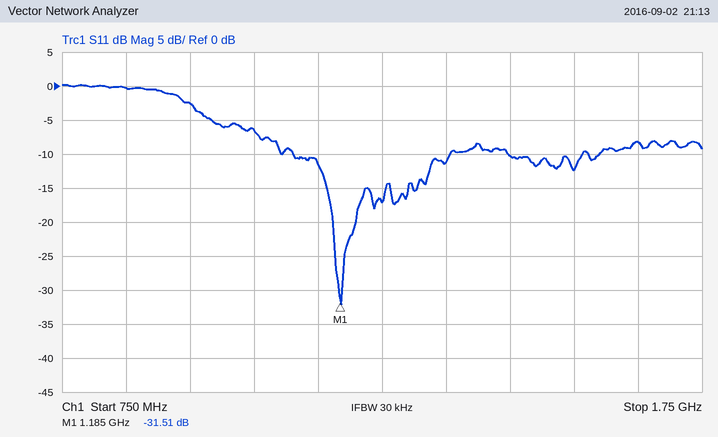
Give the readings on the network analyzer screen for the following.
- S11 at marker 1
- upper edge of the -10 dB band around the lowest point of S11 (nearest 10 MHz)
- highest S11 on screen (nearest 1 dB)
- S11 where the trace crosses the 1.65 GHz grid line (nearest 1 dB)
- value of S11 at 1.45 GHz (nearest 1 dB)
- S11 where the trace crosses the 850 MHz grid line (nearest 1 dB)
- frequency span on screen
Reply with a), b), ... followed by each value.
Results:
a) -31.51 dB
b) 1.36 GHz
c) 0 dB
d) -8 dB
e) -10 dB
f) 0 dB
g) 1 GHz
